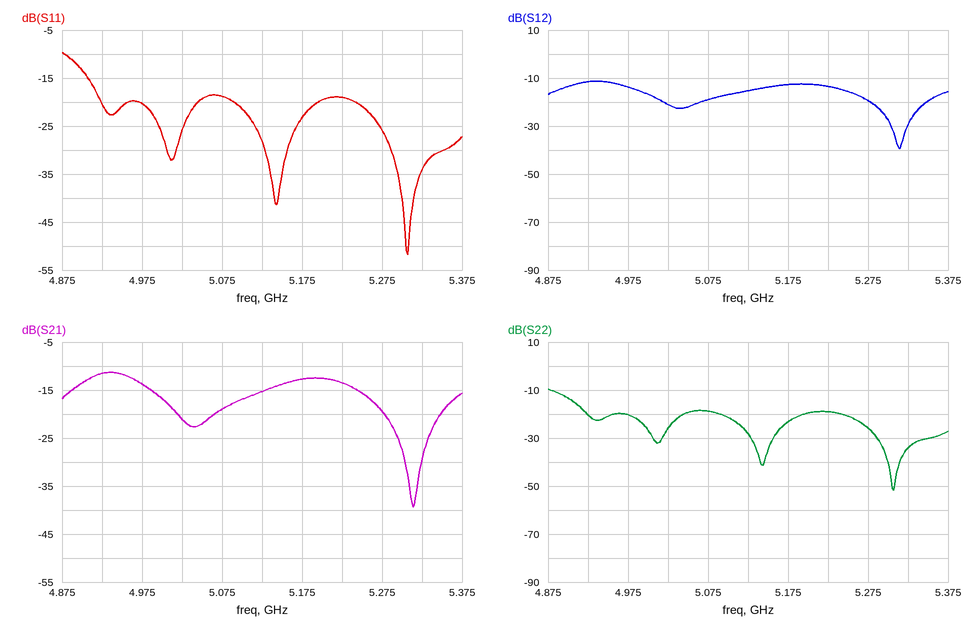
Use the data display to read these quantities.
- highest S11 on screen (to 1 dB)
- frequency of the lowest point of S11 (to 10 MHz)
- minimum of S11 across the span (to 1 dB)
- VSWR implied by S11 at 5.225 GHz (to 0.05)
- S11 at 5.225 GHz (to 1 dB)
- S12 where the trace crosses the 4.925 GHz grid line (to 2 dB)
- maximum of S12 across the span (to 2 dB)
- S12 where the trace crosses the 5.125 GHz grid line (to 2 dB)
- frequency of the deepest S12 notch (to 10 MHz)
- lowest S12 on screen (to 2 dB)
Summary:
-10 dB
5.31 GHz
-52 dB
1.25
-19 dB
-12 dB
-12 dB
-16 dB
5.31 GHz
-40 dB
